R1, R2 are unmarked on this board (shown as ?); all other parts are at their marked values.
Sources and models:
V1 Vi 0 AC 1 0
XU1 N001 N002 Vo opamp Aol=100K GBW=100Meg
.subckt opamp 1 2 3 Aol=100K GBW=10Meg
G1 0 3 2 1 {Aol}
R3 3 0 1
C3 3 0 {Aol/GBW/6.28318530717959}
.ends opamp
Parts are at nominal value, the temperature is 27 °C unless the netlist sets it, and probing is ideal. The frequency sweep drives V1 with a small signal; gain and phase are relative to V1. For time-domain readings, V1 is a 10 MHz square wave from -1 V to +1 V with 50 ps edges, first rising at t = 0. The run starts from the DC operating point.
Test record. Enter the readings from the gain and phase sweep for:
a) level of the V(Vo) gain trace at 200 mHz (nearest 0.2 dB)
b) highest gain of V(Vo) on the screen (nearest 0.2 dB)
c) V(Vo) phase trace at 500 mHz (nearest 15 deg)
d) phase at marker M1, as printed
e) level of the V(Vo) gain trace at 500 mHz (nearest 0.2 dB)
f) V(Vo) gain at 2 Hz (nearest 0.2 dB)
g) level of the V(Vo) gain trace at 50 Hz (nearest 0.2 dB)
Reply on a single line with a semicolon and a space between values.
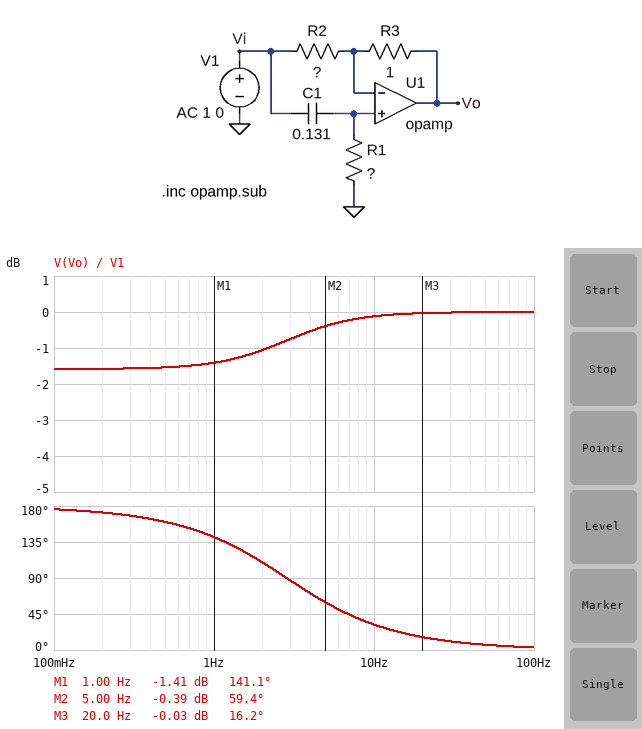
-1.6 dB; 0 dB; 165 deg; 141.1 deg; -1.6 dB; -1.0 dB; 0 dB
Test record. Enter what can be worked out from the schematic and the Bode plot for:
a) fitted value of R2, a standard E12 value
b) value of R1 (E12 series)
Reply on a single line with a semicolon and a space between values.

1.2 Ω; 0.39 Ω
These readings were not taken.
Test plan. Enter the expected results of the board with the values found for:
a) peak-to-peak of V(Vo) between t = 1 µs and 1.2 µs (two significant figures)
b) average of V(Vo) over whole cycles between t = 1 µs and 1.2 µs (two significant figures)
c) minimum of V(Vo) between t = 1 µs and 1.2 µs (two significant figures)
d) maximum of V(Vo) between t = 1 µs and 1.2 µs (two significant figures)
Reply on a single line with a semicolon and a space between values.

2.0 V; 1.8 V; 830 mV; 2.8 V
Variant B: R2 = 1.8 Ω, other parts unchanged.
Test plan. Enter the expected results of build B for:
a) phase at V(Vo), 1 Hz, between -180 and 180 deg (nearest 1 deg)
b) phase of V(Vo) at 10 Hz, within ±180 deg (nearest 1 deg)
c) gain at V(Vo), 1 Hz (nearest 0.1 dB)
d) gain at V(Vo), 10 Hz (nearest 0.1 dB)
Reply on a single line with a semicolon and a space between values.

132 deg; 27 deg; -4.3 dB; -0.3 dB
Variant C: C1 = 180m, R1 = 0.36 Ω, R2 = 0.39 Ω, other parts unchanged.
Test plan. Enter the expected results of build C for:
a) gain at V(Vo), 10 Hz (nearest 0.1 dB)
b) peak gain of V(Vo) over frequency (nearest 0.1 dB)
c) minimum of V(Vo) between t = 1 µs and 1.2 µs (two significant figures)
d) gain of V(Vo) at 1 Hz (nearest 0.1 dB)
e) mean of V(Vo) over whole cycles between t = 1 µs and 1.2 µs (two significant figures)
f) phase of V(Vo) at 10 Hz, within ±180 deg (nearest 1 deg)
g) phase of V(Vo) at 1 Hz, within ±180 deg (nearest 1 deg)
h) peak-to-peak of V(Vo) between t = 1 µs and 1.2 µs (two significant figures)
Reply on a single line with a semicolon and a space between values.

1.2 dB; 8.2 dB; 2.6 V; 7.6 dB; 3.6 V; 46 deg; 149 deg; 2.0 V
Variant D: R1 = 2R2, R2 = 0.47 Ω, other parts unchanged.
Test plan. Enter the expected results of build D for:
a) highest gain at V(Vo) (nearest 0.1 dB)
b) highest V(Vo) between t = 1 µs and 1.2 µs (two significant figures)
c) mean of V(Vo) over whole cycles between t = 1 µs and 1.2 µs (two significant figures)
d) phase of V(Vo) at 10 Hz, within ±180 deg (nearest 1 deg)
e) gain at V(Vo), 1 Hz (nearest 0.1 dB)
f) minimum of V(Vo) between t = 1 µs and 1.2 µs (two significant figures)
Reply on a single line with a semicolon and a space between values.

6.6 dB; 4.1 V; 3.1 V; 10 deg; 2.6 dB; 2.1 V
